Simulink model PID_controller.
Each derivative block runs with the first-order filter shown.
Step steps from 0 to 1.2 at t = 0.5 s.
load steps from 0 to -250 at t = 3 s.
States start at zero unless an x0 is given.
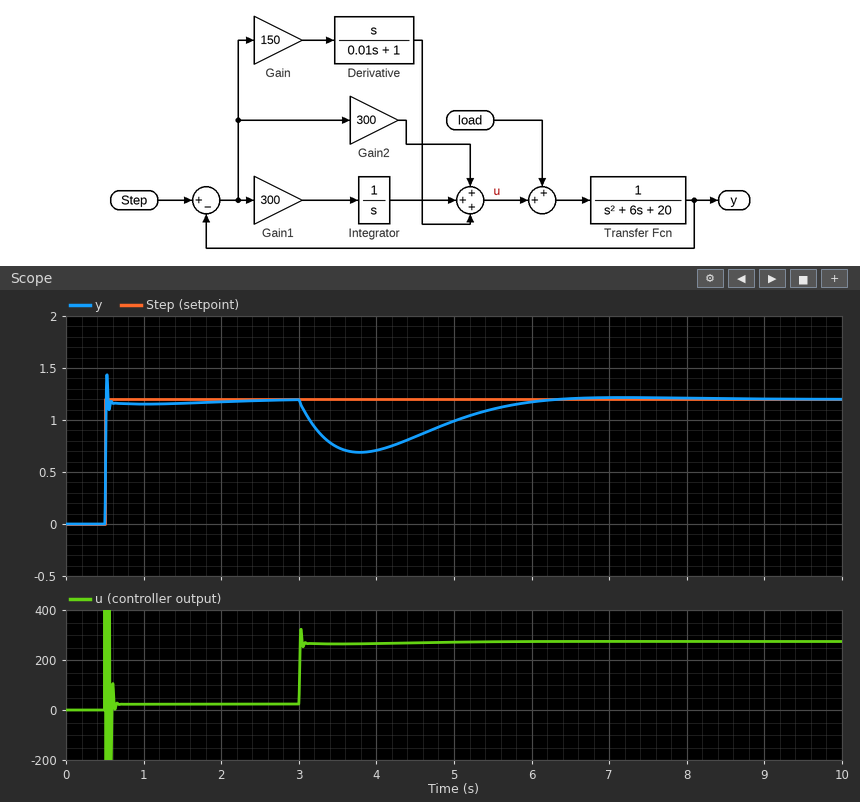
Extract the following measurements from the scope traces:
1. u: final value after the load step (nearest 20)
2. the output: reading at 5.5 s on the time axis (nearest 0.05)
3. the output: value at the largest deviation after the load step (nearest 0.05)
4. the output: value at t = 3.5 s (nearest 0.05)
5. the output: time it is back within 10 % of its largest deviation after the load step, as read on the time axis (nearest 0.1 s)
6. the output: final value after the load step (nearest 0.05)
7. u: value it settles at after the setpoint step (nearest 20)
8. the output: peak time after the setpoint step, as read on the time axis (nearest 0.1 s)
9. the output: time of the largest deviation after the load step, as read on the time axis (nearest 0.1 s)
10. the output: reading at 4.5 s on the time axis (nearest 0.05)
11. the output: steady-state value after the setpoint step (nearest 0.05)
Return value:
280
1.10
0.70
0.75
5.8 s
1.20
20
0.5 s
3.8 s
0.85
1.20
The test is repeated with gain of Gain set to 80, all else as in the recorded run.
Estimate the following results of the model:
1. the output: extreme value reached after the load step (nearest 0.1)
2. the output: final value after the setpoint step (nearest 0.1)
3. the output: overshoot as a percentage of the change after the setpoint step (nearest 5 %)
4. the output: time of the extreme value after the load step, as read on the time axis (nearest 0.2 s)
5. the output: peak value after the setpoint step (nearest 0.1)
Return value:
0.6
1.2
10 %
3.6 s
1.3
